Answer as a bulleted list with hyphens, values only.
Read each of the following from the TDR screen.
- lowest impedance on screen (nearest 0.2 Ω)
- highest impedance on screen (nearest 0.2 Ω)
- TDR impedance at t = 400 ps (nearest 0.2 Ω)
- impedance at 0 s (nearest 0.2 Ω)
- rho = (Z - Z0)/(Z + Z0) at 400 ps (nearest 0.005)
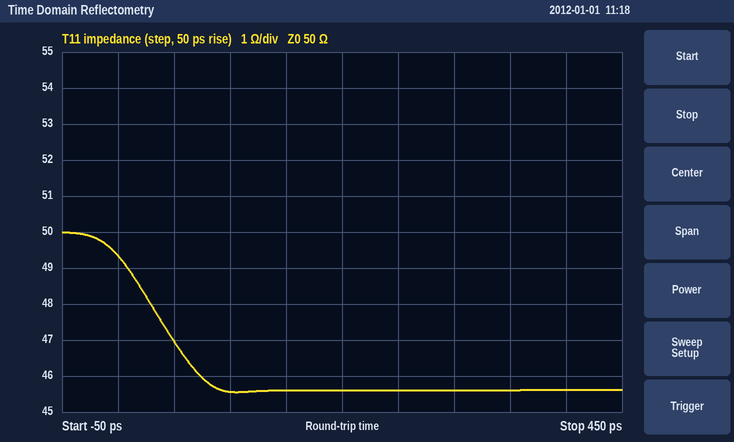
- 45.6 Ω
- 50.0 Ω
- 45.6 Ω
- 49.4 Ω
- -0.045
